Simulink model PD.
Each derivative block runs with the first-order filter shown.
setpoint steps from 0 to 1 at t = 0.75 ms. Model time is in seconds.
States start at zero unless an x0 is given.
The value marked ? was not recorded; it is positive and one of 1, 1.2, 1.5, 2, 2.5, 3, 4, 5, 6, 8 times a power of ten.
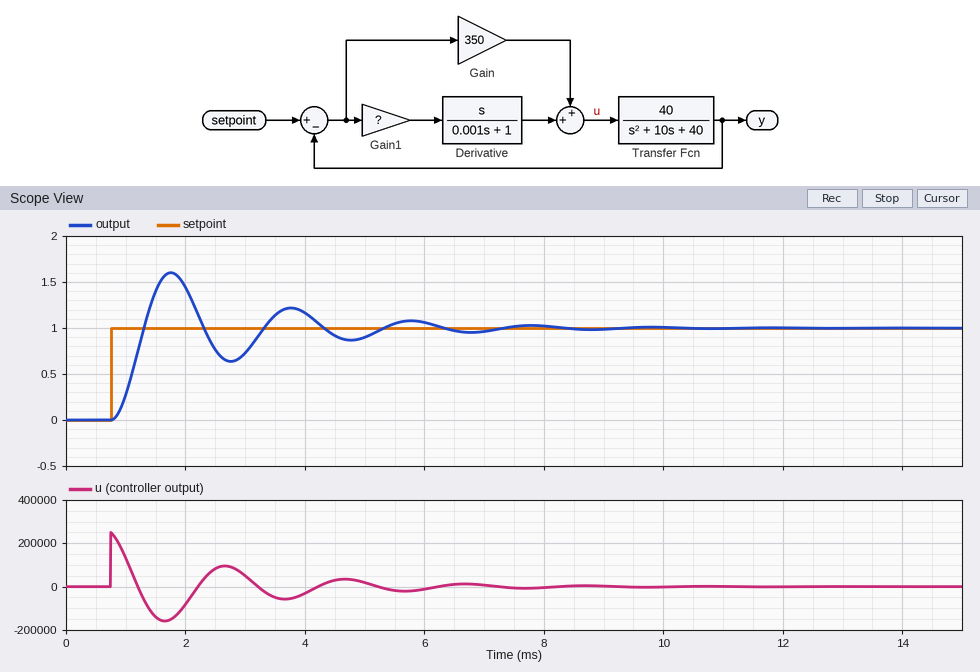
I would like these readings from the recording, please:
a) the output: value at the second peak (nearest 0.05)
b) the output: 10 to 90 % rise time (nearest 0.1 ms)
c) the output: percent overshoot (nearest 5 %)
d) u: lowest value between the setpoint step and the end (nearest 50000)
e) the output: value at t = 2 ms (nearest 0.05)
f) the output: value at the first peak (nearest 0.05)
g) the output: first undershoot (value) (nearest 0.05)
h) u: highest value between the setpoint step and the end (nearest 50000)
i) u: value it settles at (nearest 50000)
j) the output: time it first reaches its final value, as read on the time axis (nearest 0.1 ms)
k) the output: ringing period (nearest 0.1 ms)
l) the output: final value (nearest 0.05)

1.20
0.4 ms
60 %
-150000
1.45
1.60
0.65
250000
0
1.3 ms
2.0 ms
1.00
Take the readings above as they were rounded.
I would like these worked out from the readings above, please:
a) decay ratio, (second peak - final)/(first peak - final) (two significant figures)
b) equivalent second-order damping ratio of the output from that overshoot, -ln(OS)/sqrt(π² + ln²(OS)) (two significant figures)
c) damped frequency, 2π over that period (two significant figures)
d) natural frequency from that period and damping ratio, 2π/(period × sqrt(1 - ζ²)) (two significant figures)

0.33
0.16
3.1 rad/ms
3.2 rad/ms
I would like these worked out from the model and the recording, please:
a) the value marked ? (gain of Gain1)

250
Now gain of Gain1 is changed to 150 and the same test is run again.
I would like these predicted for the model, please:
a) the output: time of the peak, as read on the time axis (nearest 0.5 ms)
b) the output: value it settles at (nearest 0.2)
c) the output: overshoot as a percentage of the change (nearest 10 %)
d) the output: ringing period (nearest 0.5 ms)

2.0 ms
1.0
50 %
2.5 ms
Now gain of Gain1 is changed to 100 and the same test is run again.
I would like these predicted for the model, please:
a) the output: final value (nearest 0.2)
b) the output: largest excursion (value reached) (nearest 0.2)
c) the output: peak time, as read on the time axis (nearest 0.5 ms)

1.0
1.4
2.5 ms
